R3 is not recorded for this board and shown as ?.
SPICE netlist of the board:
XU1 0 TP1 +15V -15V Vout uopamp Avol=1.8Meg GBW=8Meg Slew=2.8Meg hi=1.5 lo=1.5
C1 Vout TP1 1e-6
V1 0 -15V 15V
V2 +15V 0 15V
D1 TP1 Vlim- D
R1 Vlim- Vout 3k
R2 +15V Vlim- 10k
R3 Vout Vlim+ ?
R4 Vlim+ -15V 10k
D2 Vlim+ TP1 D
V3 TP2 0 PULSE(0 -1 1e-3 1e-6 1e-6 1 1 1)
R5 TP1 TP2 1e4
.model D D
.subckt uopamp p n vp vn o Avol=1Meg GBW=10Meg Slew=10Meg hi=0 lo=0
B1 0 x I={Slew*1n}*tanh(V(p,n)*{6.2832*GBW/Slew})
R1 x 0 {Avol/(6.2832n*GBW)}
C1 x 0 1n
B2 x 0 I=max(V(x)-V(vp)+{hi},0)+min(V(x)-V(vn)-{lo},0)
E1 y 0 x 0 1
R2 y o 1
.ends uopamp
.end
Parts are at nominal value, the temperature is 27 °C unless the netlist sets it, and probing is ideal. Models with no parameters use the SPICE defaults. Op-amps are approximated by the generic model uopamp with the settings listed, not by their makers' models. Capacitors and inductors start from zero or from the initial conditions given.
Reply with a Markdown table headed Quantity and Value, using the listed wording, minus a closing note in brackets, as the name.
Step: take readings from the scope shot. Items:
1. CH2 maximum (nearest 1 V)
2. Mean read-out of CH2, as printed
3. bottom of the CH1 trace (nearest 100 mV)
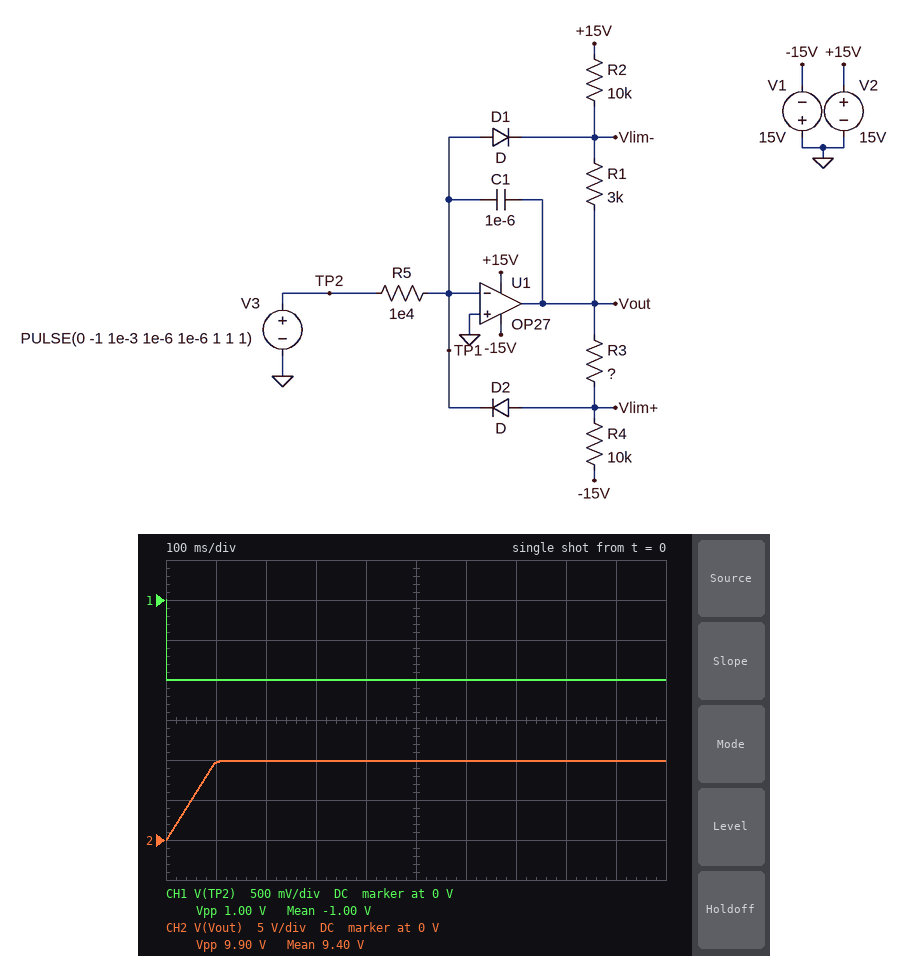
| Quantity | Value |
|---|---|
| CH2 maximum | 10 V |
| Mean read-out of CH2, as printed | 9.40 V |
| bottom of the CH1 trace | -1.0 V |
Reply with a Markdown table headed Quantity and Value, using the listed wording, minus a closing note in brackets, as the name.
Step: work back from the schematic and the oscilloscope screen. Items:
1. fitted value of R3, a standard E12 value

| Quantity | Value |
|---|---|
| fitted value of R3, a standard E12 value | 5.6 kΩ |
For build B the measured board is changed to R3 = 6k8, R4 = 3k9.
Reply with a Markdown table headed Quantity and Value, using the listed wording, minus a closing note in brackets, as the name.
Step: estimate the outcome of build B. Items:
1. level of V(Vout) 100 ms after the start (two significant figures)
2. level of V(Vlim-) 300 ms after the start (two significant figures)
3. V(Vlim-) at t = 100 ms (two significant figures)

| Quantity | Value |
|---|---|
| level of V(Vout) 100 ms after the start | 9.9 V |
| level of V(Vlim-) 300 ms after the start | 14 V |
| V(Vlim-) at t = 100 ms | 11 V |
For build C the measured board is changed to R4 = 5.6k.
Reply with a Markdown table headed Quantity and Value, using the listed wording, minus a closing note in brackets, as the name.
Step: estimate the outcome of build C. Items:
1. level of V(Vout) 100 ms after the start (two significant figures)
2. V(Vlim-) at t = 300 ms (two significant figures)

| Quantity | Value |
|---|---|
| level of V(Vout) 100 ms after the start | 9.9 V |
| V(Vlim-) at t = 300 ms | 14 V |
